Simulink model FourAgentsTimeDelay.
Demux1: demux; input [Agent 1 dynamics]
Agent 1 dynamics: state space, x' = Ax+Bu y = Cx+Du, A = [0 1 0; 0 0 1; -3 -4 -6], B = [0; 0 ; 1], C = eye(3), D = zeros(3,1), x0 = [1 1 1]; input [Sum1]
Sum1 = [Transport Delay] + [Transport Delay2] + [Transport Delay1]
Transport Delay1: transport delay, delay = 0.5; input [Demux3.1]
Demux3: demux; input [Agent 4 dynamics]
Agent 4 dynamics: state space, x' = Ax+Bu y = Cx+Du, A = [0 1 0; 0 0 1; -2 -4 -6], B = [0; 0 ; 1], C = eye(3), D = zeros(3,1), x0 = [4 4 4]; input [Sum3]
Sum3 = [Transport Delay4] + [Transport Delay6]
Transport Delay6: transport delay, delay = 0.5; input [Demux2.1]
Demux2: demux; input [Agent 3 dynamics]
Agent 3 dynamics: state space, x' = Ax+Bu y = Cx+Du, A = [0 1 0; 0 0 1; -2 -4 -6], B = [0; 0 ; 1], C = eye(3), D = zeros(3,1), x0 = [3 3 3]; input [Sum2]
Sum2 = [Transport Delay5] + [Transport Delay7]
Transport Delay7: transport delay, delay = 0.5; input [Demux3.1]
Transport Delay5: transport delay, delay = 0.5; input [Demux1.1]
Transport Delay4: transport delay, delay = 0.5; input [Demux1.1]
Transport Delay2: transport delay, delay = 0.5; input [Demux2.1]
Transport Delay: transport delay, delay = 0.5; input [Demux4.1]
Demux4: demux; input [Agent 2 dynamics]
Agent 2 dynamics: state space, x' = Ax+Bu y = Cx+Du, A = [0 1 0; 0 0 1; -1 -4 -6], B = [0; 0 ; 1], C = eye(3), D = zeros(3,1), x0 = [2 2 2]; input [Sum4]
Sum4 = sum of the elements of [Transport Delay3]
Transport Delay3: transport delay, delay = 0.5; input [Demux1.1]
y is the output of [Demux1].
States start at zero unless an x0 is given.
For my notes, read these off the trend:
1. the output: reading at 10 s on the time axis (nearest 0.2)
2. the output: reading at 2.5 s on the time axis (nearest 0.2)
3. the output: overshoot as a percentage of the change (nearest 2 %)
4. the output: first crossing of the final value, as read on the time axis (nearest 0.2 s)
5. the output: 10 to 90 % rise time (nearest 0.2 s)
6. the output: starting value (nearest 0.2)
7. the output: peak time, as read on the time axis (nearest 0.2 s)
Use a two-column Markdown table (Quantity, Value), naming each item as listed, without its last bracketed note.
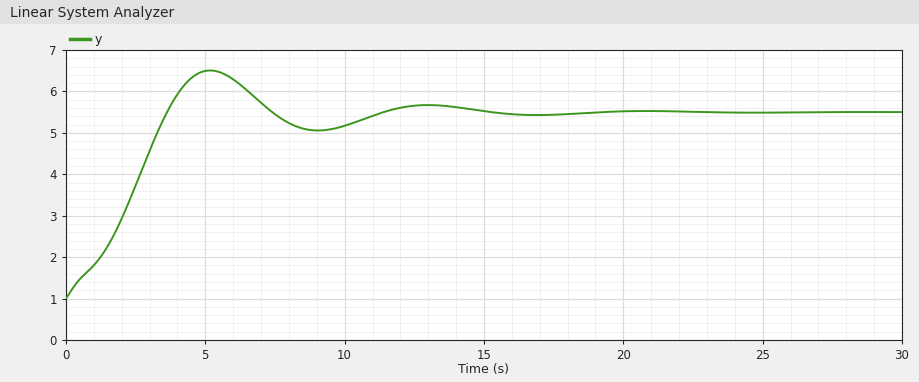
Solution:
| Quantity | Value |
|---|---|
| the output: reading at 10 s on the time axis | 5.2 |
| the output: reading at 2.5 s on the time axis | 3.8 |
| the output: overshoot as a percentage of the change | 22 % |
| the output: first crossing of the final value, as read on the time axis | 3.6 s |
| the output: 10 to 90 % rise time | 2.8 s |
| the output: starting value | 1.0 |
| the output: peak time, as read on the time axis | 5.2 s |
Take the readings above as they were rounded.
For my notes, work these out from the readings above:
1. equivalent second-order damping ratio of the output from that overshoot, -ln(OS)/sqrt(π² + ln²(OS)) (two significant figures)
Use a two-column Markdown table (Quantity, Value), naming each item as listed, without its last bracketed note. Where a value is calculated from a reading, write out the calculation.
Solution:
| Quantity | Value |
|---|---|
| equivalent second-order damping ratio of the output from that overshoot, -ln(OS)/sqrt(π² + ln²(OS)) | ln(0.22) = -1.514; 1.514 / sqrt(9.870 + 2.293) = 0.43 |
